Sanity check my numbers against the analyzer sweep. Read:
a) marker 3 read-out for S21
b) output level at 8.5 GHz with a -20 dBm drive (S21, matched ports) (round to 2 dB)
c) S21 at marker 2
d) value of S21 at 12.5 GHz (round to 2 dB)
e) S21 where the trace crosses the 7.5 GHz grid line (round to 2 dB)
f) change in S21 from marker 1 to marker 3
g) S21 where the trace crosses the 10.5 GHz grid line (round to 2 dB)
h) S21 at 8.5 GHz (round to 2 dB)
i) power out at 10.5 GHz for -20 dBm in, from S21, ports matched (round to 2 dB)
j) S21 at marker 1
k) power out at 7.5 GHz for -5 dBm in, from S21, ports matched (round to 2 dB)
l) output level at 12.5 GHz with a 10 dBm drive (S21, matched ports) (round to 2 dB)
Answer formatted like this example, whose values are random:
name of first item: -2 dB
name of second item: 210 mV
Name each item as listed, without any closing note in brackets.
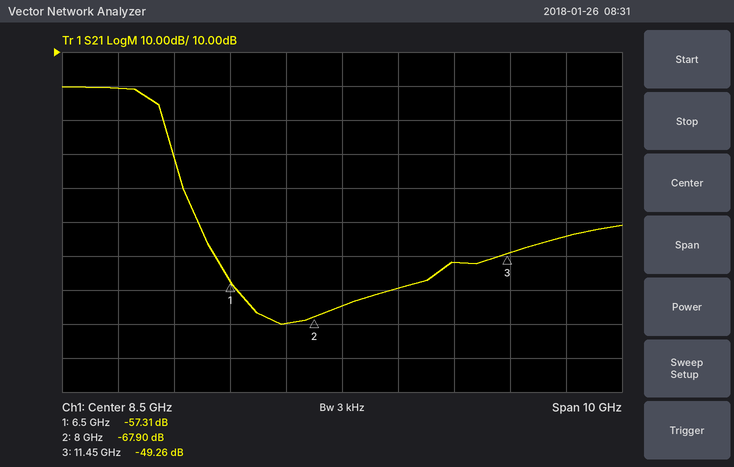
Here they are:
marker 3 read-out for S21: -49.26 dB
output level at 8.5 GHz with a -20 dBm drive (S21, matched ports): -84 dBm
S21 at marker 2: -67.90 dB
value of S21 at 12.5 GHz: -44 dB
S21 where the trace crosses the 7.5 GHz grid line: -70 dB
change in S21 from marker 1 to marker 3: 8.05 dB
S21 where the trace crosses the 10.5 GHz grid line: -52 dB
S21 at 8.5 GHz: -64 dB
power out at 10.5 GHz for -20 dBm in, from S21, ports matched: -72 dBm
S21 at marker 1: -57.31 dB
power out at 7.5 GHz for -5 dBm in, from S21, ports matched: -74 dBm
output level at 12.5 GHz with a 10 dBm drive (S21, matched ports): -34 dBm
